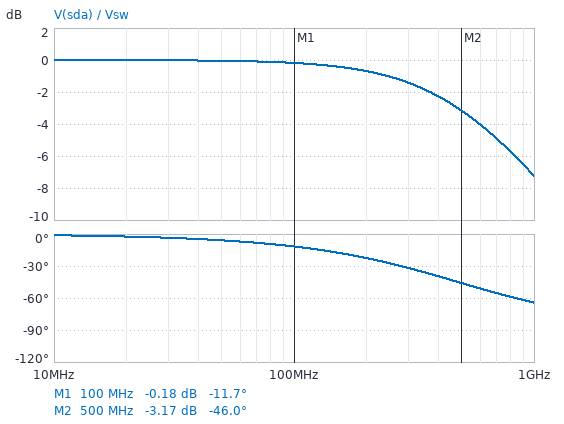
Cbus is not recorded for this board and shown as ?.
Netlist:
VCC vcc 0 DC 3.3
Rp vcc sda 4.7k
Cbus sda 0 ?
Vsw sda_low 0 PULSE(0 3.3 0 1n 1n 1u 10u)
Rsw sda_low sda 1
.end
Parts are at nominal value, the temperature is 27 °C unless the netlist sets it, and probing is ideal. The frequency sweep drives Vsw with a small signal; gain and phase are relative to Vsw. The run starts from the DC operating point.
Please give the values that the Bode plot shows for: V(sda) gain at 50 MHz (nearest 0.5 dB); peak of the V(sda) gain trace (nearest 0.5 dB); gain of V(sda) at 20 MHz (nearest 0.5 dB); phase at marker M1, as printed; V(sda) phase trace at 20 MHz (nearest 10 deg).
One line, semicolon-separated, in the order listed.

0 dB; 0 dB; 0 dB; -11.7 deg; 0 deg
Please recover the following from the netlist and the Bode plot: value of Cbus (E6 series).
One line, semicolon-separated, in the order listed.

330 pF
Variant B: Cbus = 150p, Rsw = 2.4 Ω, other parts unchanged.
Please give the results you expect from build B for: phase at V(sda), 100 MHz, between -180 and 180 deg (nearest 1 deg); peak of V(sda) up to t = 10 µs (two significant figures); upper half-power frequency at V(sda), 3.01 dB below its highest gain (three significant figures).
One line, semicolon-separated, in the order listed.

-13 deg; 3.3 V; 442 MHz
